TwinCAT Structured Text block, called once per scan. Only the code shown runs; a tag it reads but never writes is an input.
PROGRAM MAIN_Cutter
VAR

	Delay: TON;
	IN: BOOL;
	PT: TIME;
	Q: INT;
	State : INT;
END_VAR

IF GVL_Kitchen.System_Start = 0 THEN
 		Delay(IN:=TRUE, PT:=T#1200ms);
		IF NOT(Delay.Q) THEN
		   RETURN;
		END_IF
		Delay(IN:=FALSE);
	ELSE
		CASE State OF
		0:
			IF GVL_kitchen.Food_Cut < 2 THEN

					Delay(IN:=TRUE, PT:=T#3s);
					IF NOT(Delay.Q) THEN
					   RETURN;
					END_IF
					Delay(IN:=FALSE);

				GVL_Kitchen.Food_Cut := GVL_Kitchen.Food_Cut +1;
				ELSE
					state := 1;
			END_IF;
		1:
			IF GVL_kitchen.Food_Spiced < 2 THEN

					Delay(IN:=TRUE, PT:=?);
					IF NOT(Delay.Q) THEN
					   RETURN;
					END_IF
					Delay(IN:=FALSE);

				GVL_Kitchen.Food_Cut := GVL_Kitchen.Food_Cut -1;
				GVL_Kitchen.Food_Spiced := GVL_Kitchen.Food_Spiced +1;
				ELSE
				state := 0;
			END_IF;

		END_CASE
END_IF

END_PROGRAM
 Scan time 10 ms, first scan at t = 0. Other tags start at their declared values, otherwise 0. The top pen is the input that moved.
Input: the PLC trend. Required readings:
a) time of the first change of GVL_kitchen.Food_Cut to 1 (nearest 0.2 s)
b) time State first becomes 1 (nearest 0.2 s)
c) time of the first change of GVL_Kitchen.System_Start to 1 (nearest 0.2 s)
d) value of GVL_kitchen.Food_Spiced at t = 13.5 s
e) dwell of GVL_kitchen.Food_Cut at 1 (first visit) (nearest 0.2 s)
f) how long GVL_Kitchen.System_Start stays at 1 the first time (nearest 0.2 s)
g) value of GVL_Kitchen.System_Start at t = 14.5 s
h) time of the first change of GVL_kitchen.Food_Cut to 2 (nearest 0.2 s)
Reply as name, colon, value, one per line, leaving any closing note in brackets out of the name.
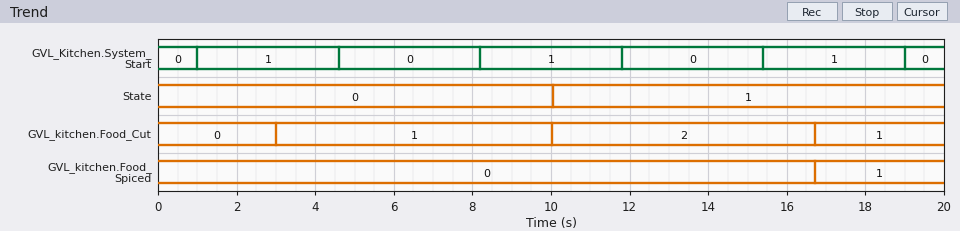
time of the first change of GVL_kitchen.Food_Cut to 1: 3.0 s
time State first becomes 1: 10.0 s
time of the first change of GVL_Kitchen.System_Start to 1: 1.0 s
value of GVL_kitchen.Food_Spiced at t = 13.5 s: 0
dwell of GVL_kitchen.Food_Cut at 1 (first visit): 7.0 s
how long GVL_Kitchen.System_Start stays at 1 the first time: 3.6 s
value of GVL_Kitchen.System_Start at t = 14.5 s: 0
time of the first change of GVL_kitchen.Food_Cut to 2: 10.0 s
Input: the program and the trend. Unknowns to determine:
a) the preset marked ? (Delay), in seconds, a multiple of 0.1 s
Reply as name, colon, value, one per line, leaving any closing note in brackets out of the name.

the preset marked ? (Delay), in seconds, a multiple of 0.1 s: 2.5 s
